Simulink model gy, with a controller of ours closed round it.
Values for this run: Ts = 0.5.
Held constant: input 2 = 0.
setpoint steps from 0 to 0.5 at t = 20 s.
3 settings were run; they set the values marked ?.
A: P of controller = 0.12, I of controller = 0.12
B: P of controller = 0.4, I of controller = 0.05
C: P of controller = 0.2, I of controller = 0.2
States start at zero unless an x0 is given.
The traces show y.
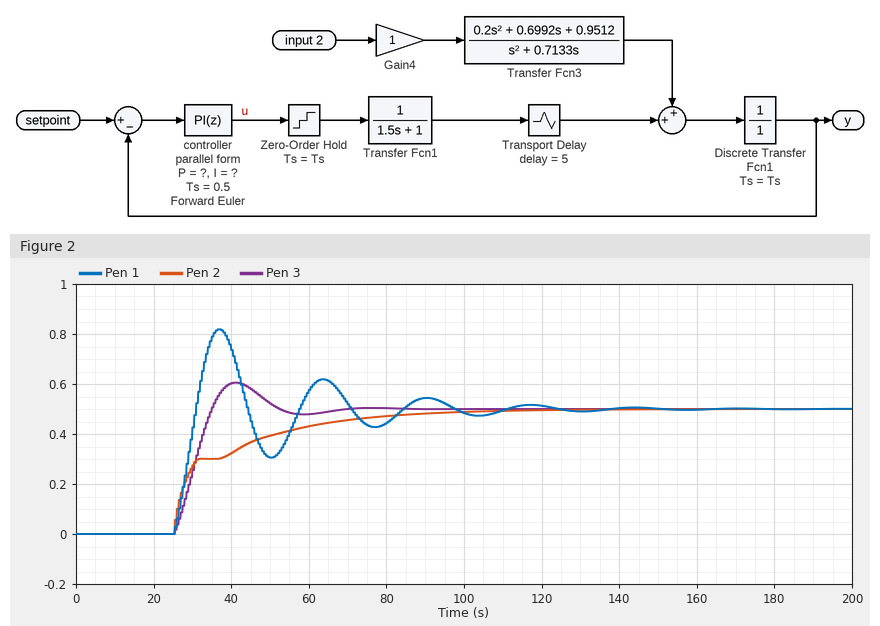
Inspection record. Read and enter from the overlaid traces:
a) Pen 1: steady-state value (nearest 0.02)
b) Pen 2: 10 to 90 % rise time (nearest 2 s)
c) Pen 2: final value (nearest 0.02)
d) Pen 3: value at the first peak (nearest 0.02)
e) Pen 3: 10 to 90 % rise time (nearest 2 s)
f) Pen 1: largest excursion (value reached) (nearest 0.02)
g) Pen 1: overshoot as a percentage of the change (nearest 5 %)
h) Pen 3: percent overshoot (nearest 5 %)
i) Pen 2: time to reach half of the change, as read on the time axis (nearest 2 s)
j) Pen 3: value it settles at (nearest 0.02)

0.50
42 s
0.50
0.60
8 s
0.82
65 %
20 %
30 s
0.50
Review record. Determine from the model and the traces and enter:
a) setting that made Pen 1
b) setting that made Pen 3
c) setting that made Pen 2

C
A
B
